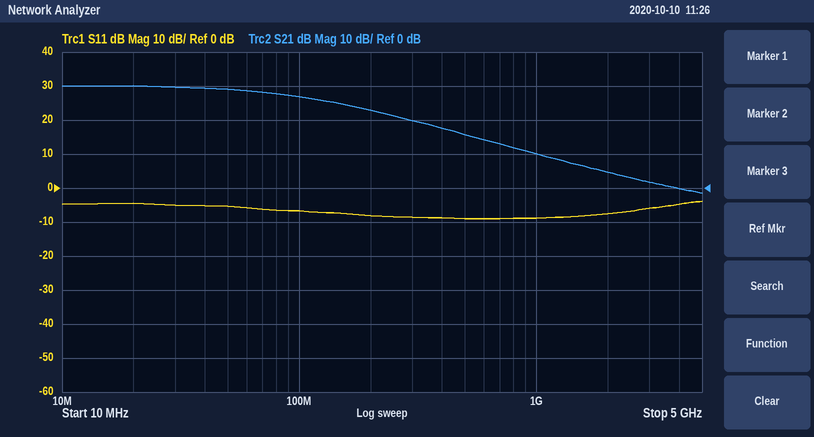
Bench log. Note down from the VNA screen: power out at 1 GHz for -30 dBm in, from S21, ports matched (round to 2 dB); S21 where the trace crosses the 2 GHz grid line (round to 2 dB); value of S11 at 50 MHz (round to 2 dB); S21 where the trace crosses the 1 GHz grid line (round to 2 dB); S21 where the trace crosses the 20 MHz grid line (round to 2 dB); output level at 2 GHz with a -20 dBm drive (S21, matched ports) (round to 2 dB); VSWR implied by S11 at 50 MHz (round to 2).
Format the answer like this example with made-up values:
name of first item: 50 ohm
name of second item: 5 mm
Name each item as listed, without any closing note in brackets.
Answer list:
power out at 1 GHz for -30 dBm in, from S21, ports matched: -20 dBm
S21 where the trace crosses the 2 GHz grid line: 4 dB
value of S11 at 50 MHz: -6 dB
S21 where the trace crosses the 1 GHz grid line: 10 dB
S21 where the trace crosses the 20 MHz grid line: 30 dB
output level at 2 GHz with a -20 dBm drive (S21, matched ports): -16 dBm
VSWR implied by S11 at 50 MHz: 4
